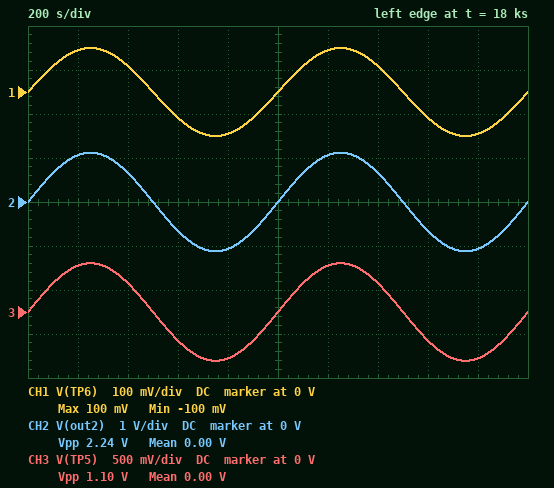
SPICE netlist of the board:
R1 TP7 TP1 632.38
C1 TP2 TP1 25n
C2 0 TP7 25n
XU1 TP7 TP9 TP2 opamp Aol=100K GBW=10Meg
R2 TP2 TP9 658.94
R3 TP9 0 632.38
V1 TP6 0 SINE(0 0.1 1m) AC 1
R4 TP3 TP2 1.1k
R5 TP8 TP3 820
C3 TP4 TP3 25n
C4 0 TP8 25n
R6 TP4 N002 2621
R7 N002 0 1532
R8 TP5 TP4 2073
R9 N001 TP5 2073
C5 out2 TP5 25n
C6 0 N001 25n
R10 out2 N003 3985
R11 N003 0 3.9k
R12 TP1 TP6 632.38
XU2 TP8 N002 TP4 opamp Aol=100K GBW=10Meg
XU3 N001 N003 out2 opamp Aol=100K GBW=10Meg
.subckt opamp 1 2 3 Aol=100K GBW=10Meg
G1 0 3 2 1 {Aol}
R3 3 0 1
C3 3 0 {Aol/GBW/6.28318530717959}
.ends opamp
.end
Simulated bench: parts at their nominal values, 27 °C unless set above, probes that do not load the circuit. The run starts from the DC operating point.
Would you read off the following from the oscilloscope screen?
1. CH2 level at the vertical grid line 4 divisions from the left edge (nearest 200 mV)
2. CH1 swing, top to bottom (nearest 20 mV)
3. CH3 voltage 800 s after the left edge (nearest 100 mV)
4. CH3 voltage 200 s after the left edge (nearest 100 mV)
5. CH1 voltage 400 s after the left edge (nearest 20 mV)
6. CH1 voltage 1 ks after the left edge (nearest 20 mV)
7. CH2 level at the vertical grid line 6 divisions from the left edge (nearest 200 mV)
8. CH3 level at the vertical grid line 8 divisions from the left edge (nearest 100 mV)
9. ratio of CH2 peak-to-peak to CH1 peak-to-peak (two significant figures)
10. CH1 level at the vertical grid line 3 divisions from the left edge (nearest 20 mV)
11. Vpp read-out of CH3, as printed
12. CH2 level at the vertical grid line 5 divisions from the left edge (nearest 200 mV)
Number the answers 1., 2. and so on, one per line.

1. -1.0 V
2. 200 mV
3. -500 mV
4. 500 mV
5. 60 mV
6. 0 V
7. 1.0 V
8. -300 mV
9. 11
10. -60 mV
11. 1.10 V
12. 0 V
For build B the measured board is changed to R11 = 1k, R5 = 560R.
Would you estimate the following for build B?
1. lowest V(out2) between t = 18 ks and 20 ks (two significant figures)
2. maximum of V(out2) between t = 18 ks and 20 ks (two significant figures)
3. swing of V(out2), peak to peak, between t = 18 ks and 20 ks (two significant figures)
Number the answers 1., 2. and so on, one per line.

1. -2.8 V
2. 2.8 V
3. 5.5 V
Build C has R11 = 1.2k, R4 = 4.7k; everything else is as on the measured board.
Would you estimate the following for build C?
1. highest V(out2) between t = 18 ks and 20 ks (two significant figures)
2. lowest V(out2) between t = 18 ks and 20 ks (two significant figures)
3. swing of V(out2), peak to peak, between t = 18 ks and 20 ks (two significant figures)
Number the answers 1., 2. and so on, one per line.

1. 2.4 V
2. -2.4 V
3. 4.8 V
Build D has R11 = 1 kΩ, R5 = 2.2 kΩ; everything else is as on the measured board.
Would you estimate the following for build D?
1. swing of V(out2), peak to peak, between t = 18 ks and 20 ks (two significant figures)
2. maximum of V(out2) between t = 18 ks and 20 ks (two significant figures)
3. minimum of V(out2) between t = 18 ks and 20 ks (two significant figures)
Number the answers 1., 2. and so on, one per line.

1. 5.5 V
2. 2.8 V
3. -2.8 V
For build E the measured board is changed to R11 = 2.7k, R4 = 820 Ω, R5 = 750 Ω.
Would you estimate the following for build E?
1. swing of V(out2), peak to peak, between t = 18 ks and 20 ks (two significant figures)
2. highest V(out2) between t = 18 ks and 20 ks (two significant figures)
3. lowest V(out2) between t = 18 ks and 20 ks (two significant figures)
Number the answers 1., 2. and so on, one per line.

1. 2.7 V
2. 1.4 V
3. -1.4 V
